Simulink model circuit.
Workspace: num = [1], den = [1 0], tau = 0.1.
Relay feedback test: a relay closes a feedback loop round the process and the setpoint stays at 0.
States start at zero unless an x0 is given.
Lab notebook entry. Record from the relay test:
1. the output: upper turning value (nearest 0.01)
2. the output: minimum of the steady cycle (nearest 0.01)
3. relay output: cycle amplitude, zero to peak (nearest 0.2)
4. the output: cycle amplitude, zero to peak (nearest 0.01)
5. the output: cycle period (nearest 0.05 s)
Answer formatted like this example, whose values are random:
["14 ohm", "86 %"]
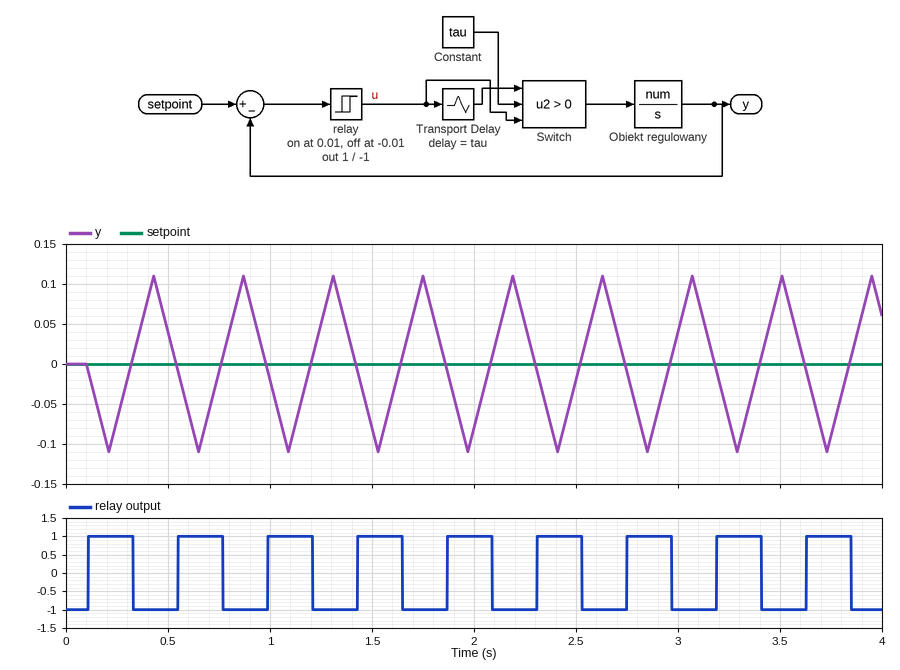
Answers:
["0.11", "-0.11", "1.0", "0.11", "0.45 s"]
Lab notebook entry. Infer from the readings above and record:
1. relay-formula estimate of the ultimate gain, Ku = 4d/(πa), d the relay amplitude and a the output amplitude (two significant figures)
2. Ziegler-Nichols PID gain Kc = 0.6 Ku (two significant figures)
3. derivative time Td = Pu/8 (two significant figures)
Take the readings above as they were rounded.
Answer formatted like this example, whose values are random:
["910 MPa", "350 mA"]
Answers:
["12", "7.2", "0.056 s"]
